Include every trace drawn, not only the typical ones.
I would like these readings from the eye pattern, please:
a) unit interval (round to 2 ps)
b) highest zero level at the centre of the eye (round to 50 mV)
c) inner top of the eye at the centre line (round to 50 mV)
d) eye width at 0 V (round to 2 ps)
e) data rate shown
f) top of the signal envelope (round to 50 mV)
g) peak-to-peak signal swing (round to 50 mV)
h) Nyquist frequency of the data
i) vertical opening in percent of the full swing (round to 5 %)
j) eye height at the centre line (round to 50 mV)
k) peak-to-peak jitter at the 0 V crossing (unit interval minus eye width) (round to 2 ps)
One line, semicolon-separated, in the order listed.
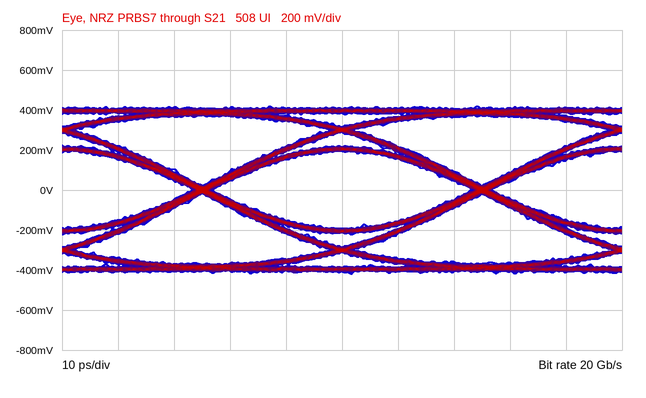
50 ps; -200 mV; 200 mV; 46 ps; 20 Gb/s; 400 mV; 850 mV; 10 GHz; 45 %; 400 mV; 4 ps
